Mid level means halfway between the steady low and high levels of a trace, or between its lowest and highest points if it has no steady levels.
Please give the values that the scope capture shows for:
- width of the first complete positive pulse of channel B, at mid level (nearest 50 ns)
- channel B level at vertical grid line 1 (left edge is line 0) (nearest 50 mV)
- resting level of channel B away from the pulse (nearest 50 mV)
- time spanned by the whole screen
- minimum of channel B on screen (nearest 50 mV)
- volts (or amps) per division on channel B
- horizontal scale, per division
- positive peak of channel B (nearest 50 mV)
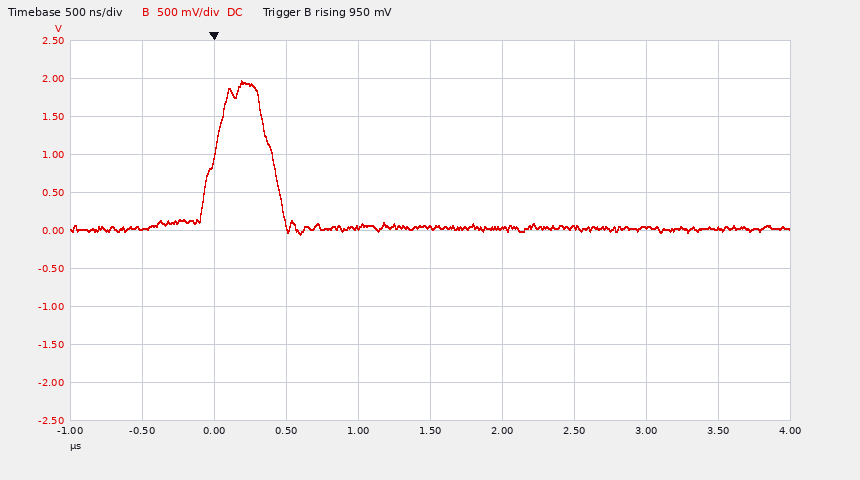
400 ns
0 mV
50 mV
5 µs
-50 mV
500 mV
500 ns
1.95 V
